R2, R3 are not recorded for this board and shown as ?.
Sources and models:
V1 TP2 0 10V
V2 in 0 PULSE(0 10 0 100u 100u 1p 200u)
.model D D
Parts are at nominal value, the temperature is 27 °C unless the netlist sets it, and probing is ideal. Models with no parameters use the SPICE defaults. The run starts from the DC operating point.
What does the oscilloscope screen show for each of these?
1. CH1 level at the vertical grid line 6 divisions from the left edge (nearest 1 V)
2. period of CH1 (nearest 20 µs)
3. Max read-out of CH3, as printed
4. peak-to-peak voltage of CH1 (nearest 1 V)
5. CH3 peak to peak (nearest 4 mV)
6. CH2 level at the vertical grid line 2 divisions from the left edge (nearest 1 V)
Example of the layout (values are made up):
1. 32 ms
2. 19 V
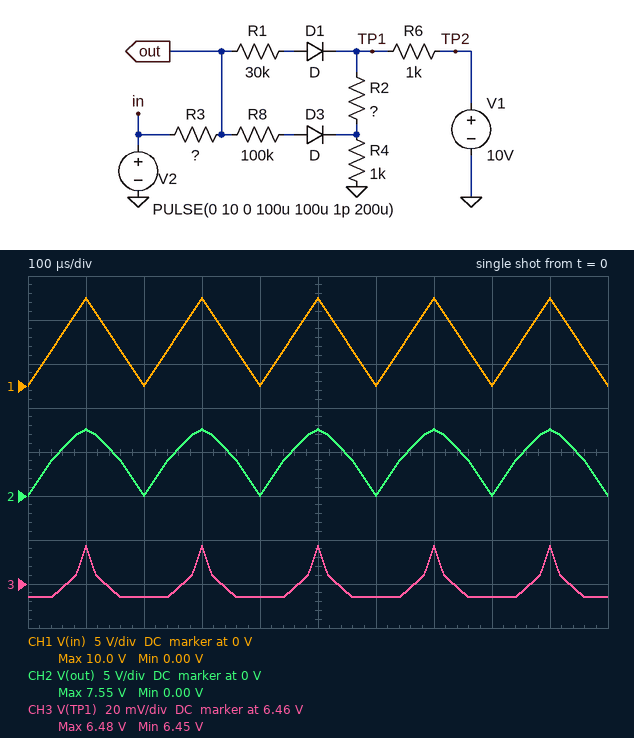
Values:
1. 0 V
2. 200 µs
3. 6.48 V
4. 10 V
5. 24 mV
6. 0 V
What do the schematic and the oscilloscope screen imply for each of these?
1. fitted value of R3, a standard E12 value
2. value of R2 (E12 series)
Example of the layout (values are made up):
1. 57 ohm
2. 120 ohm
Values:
1. 47 kΩ
2. 820 Ω
